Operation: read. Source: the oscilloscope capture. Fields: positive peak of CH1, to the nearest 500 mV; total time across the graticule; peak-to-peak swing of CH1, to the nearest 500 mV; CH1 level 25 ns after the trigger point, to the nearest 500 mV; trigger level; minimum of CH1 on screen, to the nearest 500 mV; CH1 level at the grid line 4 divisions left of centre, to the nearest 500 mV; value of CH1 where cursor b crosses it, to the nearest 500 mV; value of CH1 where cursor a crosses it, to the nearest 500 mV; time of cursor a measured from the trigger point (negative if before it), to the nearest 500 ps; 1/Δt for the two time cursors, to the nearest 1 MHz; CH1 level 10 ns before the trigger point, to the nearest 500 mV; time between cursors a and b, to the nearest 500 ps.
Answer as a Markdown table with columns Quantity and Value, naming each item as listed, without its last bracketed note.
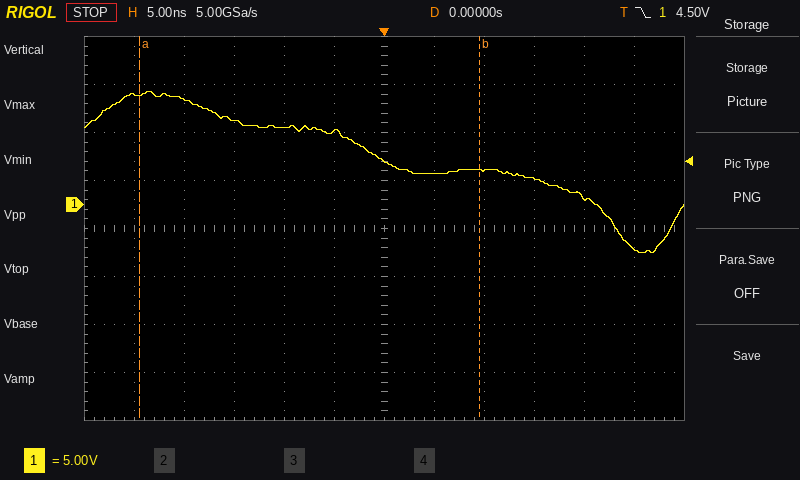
| Quantity | Value |
|---|---|
| positive peak of CH1, to the nearest 500 mV | 12.0 V |
| total time across the graticule | 60 ns |
| peak-to-peak swing of CH1, to the nearest 500 mV | 17.0 V |
| CH1 level 25 ns after the trigger point, to the nearest 500 mV | -4.5 V |
| trigger level | 4.50 V |
| minimum of CH1 on screen, to the nearest 500 mV | -5.0 V |
| CH1 level at the grid line 4 divisions left of centre, to the nearest 500 mV | 11.0 V |
| value of CH1 where cursor b crosses it, to the nearest 500 mV | 3.5 V |
| value of CH1 where cursor a crosses it, to the nearest 500 mV | 11.5 V |
| time of cursor a measured from the trigger point (negative if before it), to the nearest 500 ps | -24.5 ns |
| 1/Δt for the two time cursors, to the nearest 1 MHz | 29 MHz |
| CH1 level 10 ns before the trigger point, to the nearest 500 mV | 8.0 V |
| time between cursors a and b, to the nearest 500 ps | 34.0 ns |
